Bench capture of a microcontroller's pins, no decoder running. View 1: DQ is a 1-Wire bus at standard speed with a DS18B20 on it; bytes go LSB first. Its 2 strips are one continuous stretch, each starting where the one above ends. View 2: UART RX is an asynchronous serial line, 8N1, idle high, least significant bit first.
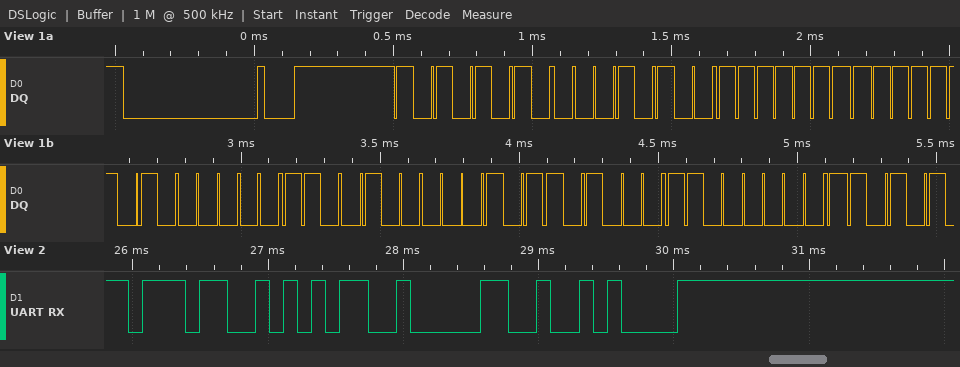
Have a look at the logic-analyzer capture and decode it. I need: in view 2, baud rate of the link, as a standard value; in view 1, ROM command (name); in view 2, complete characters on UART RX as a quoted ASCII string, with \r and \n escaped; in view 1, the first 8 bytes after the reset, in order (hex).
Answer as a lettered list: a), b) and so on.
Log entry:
a) 9600 baud
b) Match ROM
c) "750\n"
d) 55 28 FF 5F 60 82 16 03
